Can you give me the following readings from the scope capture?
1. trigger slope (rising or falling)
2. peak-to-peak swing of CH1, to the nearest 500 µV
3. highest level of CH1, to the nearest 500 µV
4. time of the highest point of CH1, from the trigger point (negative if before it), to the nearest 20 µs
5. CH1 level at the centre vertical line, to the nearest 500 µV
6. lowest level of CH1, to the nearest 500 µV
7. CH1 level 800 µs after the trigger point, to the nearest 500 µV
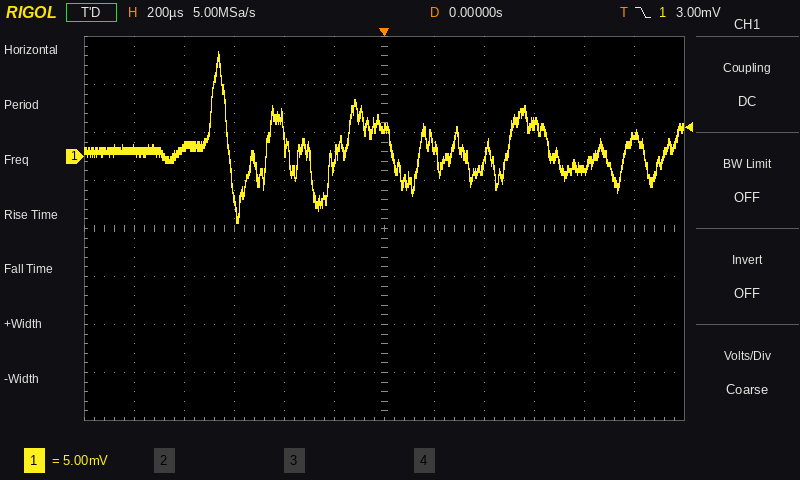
falling
18.0 mV
11.0 mV
-660 µs
3.0 mV
-7.0 mV
-1.5 mV
